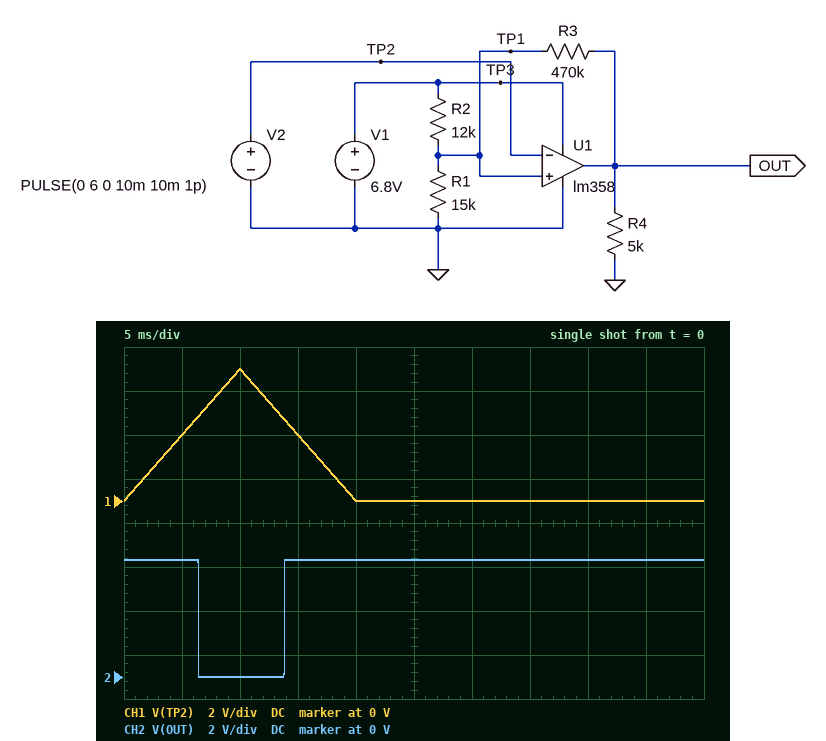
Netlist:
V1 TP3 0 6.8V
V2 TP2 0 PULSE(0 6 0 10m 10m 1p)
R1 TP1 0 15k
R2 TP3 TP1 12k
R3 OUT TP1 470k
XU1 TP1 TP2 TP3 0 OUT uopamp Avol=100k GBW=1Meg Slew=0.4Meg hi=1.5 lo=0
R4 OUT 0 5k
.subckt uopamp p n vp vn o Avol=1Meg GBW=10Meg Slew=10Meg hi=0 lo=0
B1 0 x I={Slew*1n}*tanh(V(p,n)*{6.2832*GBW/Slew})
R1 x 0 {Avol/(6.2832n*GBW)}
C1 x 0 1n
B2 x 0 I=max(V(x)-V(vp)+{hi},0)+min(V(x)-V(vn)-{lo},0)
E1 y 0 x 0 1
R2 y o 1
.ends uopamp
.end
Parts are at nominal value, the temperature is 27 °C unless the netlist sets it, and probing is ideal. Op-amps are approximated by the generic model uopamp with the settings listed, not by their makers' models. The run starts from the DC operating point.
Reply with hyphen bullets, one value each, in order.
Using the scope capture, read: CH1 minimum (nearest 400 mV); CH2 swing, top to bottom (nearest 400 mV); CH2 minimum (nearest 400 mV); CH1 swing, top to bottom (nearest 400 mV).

- 0 V
- 5.2 V
- 0 V
- 6.0 V
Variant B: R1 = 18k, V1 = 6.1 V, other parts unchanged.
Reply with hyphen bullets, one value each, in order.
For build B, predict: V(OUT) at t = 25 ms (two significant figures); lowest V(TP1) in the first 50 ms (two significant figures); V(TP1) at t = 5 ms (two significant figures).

- 4.6 V
- 3.6 V
- 3.7 V
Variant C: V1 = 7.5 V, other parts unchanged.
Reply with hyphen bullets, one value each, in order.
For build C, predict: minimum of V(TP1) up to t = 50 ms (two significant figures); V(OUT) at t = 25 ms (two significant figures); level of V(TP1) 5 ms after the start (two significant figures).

- 4.1 V
- 6.0 V
- 4.2 V
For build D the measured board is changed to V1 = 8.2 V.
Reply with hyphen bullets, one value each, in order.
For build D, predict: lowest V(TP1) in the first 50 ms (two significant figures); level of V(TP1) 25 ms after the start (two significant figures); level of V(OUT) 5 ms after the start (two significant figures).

- 4.5 V
- 4.6 V
- 6.7 V
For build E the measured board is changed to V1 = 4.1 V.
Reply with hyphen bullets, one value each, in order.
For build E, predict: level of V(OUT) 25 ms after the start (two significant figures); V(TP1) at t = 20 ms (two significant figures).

- 2.6 V
- 2.3 V
